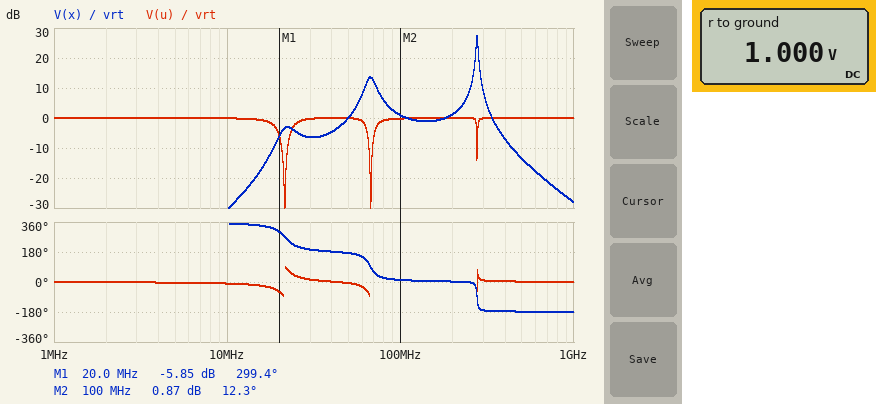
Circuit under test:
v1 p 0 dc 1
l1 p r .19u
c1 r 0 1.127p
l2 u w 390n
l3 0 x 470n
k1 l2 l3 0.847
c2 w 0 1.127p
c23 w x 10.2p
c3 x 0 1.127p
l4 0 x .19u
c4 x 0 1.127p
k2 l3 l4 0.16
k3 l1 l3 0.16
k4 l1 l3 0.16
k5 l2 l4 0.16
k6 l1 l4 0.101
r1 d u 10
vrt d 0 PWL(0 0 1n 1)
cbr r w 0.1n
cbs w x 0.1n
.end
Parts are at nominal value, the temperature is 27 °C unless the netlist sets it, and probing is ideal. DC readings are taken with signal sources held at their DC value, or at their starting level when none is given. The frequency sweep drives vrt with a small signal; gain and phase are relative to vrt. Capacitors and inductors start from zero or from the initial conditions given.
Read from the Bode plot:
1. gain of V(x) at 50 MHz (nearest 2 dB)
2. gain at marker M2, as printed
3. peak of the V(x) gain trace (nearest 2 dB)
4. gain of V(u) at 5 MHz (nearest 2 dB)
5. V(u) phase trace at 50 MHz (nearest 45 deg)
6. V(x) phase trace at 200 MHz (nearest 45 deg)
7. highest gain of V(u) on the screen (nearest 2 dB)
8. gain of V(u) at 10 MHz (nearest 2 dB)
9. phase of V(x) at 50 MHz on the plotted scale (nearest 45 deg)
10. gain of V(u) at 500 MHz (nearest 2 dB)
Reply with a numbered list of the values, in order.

1. 0 dB
2. 0.87 dB
3. 28 dB
4. 0 dB
5. 0 deg
6. 0 deg
7. 0 dB
8. 0 dB
9. 180 deg
10. 0 dB
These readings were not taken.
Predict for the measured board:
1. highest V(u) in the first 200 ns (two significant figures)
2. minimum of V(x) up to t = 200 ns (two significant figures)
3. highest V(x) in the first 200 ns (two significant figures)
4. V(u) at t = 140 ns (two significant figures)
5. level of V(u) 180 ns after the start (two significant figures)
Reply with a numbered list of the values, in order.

1. 1.1 V
2. -1.7 V
3. 1.6 V
4. 1.0 V
5. 1.0 V
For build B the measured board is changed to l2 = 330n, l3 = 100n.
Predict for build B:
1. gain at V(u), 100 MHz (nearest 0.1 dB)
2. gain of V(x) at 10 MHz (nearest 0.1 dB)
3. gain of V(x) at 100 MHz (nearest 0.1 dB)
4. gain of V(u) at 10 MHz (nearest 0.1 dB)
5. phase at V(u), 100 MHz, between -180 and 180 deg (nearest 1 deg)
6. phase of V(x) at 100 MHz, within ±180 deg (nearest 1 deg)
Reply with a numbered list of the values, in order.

1. -7.2 dB
2. -23.7 dB
3. -0.5 dB
4. -0.1 dB
5. 64 deg
6. -116 deg
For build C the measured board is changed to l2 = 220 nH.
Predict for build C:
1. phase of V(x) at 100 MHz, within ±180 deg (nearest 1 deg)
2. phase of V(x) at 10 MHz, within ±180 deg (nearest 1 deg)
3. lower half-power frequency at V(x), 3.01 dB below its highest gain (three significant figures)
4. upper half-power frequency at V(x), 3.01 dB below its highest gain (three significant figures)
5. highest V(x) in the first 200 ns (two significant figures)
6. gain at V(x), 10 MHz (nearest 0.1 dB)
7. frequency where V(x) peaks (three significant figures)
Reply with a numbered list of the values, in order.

1. 13 deg
2. 171 deg
3. 322 MHz
4. 341 MHz
5. 1.8 V
6. -53.5 dB
7. 332 MHz
